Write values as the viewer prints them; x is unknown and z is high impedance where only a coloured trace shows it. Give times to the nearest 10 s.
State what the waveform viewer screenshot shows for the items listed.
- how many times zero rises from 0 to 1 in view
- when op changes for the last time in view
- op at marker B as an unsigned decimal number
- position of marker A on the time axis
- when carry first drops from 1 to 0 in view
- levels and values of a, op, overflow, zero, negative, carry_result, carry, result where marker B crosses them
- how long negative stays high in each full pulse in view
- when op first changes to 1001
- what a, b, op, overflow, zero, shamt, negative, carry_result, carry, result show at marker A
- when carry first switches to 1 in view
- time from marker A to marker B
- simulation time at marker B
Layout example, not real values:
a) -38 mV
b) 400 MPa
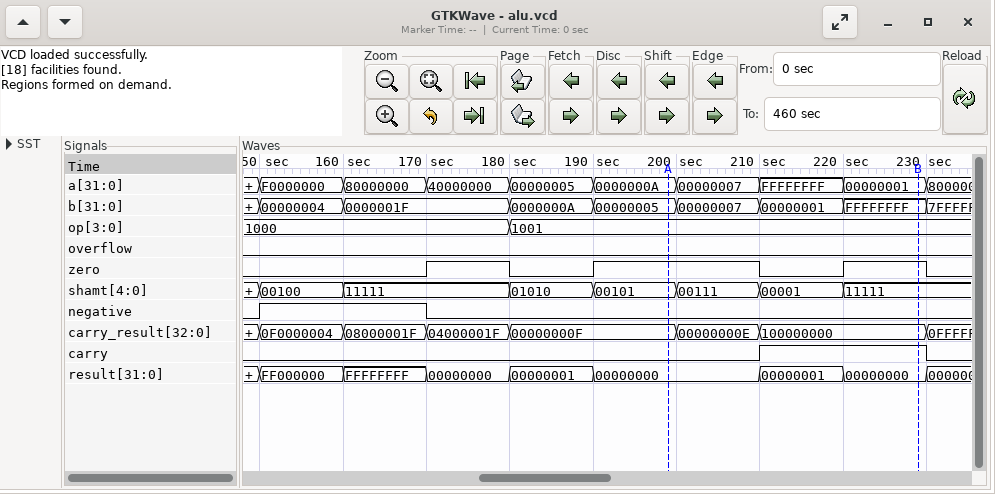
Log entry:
a) 3
b) 180 s
c) 9
d) 200 s
e) 230 s
f) a=00000001, op=1001, overflow=0, zero=1, negative=0, carry_result=100000000, carry=1, result=00000000
g) 20 s
h) 180 s
i) a=0000000A, b=00000005, op=1001, overflow=0, zero=1, shamt=00101, negative=0, carry_result=00000000F, carry=0, result=00000000
j) 210 s
k) 30 s
l) 230 s
